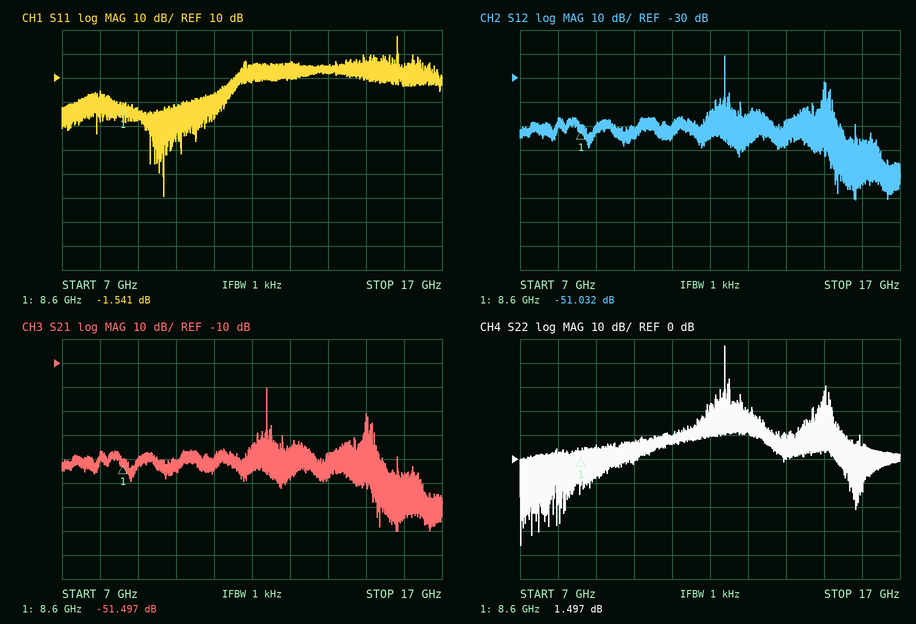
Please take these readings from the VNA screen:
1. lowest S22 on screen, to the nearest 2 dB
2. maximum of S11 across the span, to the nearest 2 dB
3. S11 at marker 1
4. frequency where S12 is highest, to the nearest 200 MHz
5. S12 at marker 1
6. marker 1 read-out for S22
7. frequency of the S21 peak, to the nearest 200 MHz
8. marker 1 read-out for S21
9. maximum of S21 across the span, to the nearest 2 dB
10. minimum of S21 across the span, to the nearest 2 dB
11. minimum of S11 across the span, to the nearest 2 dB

-36 dB
28 dB
-1.541 dB
12.4 GHz
-51.032 dB
1.497 dB
12.4 GHz
-51.497 dB
-20 dB
-80 dB
-40 dB
